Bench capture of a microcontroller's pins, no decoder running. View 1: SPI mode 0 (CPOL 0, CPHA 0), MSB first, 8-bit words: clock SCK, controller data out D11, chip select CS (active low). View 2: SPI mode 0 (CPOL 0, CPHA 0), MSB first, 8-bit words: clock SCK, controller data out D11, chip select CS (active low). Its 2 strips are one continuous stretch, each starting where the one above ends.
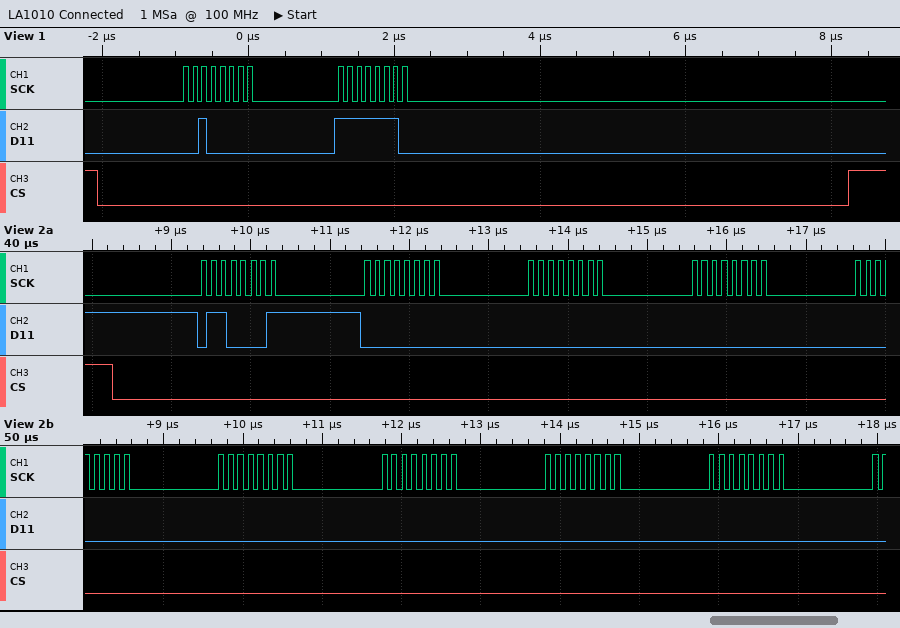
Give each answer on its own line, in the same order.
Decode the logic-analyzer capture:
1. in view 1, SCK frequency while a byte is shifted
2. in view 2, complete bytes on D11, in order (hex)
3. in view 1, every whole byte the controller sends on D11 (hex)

8 MHz
61 00 00 00 00 00 00 00 00
20 FE
